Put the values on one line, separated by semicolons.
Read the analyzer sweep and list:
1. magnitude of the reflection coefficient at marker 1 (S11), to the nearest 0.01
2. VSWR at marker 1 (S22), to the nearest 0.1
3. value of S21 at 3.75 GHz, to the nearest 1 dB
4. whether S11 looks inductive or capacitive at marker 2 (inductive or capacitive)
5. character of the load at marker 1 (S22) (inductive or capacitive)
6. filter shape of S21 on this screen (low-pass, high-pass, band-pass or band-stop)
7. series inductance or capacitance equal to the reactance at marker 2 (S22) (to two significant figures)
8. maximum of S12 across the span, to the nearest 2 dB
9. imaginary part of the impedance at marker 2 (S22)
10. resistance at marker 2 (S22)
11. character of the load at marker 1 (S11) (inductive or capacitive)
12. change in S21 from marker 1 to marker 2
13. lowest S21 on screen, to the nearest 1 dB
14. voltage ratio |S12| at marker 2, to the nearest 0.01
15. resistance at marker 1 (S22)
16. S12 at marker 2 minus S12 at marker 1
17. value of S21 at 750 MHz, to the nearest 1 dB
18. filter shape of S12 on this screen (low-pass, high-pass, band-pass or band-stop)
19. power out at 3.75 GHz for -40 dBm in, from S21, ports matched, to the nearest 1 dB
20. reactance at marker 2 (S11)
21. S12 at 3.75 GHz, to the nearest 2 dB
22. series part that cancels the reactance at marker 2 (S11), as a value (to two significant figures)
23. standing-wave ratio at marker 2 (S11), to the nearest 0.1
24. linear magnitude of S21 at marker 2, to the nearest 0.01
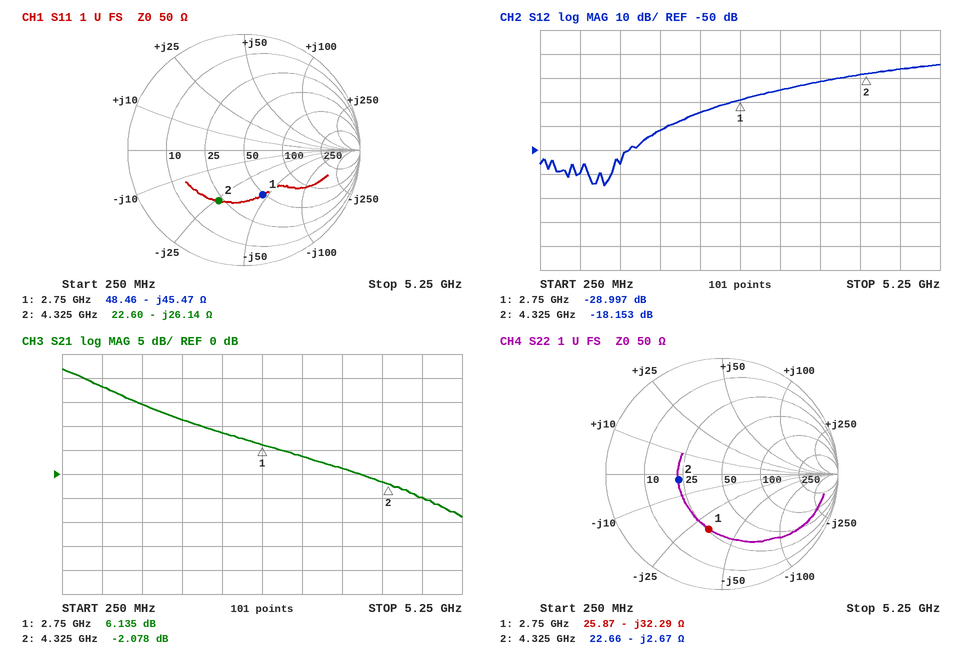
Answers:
0.42; 2.9; 1 dB; capacitive; capacitive; low-pass; 14 pF; -14 dB; -2.67 Ω; 22.66 Ω; capacitive; -8.213 dB; -9 dB; 0.12; 25.87 Ω; 10.844 dB; 18 dB; high-pass; -39 dBm; -26.14 Ω; -22 dB; 960 pH; 2.9; 0.79
